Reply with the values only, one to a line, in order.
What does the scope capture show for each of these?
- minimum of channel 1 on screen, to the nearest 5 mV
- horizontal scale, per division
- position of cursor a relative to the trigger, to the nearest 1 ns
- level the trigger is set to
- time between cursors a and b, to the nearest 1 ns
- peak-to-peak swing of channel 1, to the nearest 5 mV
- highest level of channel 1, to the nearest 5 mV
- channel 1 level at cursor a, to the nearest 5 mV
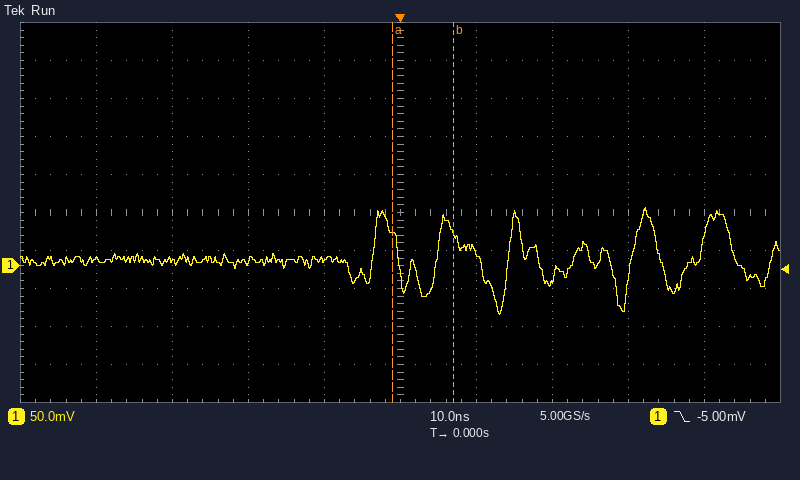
-65 mV
10 ns
-1 ns
-5.00 mV
8 ns
140 mV
75 mV
45 mV
